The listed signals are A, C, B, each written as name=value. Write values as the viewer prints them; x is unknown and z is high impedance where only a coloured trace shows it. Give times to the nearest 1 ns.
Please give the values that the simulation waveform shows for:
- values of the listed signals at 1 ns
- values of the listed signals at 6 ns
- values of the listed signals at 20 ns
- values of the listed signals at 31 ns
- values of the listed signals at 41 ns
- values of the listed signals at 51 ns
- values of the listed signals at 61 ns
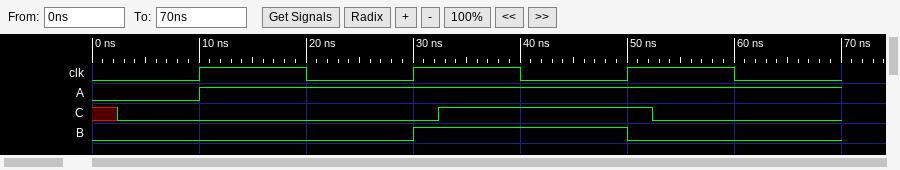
A=0, C=x, B=0
A=0, C=0, B=0
A=1, C=0, B=0
A=1, C=0, B=1
A=1, C=1, B=1
A=1, C=1, B=0
A=1, C=0, B=0
